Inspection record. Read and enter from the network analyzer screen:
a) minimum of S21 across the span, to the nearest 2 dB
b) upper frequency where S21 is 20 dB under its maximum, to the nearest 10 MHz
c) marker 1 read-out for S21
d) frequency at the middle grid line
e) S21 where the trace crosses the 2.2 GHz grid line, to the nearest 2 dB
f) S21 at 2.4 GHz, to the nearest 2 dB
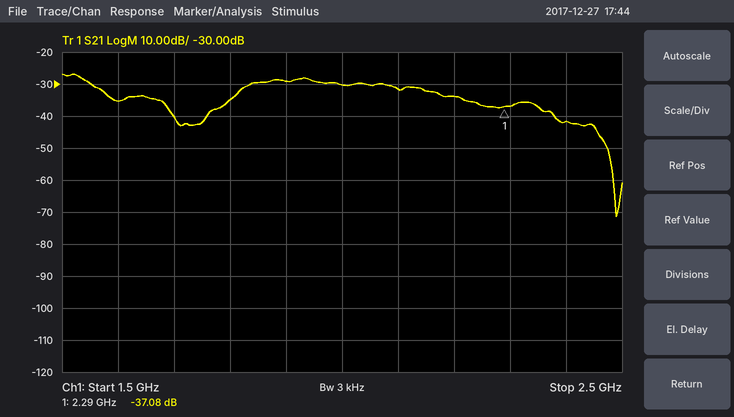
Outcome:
-72 dB
2.46 GHz
-37.08 dB
2 GHz
-34 dB
-42 dB
